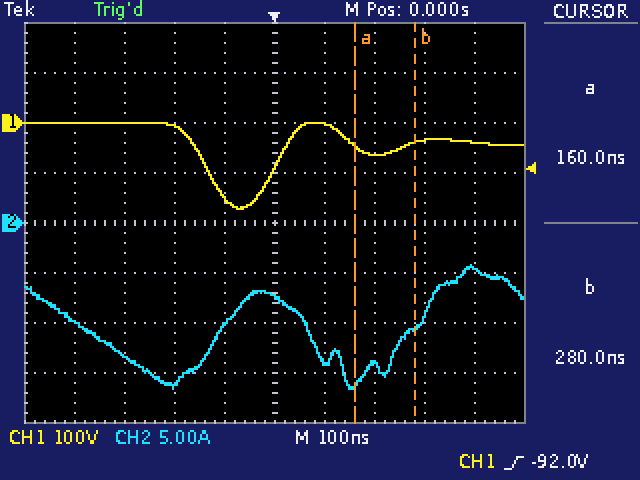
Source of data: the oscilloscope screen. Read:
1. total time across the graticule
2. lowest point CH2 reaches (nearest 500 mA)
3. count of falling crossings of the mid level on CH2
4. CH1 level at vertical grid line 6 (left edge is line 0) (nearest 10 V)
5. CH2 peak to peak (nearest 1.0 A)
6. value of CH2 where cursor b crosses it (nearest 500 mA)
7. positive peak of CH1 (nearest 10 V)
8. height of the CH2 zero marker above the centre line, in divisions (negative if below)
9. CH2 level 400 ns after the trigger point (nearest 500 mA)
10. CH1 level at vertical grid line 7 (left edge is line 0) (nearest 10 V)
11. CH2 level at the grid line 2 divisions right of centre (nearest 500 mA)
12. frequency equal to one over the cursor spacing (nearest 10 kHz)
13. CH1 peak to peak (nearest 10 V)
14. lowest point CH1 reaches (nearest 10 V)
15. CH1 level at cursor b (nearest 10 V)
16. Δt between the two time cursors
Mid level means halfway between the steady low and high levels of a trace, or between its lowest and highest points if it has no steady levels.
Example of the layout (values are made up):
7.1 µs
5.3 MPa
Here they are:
1 µs
-16.5 A
2
0 V
12.0 A
-10.5 A
0 V
0.0 div
-4.5 A
-60 V
-14.0 A
8.33 MHz
170 V
-170 V
-40 V
120 ns
